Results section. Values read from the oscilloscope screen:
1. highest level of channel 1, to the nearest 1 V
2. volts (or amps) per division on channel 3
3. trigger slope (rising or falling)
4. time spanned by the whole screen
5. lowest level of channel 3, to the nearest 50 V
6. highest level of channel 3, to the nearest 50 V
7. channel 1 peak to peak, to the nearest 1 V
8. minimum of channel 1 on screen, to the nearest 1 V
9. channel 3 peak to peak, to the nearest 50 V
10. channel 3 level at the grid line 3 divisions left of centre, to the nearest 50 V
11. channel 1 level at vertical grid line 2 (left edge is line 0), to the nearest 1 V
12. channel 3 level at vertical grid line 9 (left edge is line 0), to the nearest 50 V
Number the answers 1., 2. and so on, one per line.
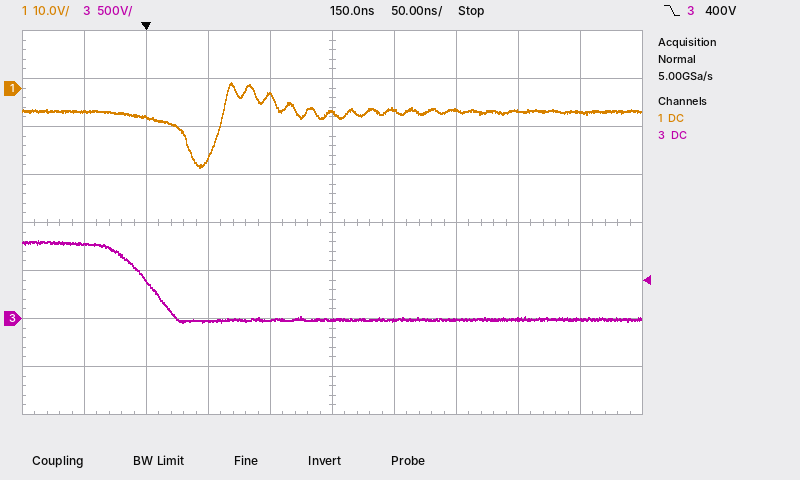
1. 1 V
2. 500 V
3. falling
4. 500 ns
5. -50 V
6. 800 V
7. 18 V
8. -17 V
9. 850 V
10. 400 V
11. -6 V
12. 0 V
